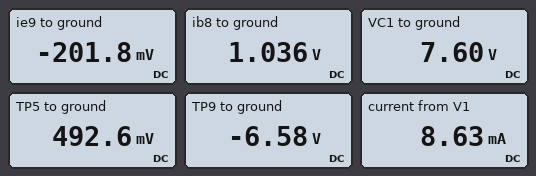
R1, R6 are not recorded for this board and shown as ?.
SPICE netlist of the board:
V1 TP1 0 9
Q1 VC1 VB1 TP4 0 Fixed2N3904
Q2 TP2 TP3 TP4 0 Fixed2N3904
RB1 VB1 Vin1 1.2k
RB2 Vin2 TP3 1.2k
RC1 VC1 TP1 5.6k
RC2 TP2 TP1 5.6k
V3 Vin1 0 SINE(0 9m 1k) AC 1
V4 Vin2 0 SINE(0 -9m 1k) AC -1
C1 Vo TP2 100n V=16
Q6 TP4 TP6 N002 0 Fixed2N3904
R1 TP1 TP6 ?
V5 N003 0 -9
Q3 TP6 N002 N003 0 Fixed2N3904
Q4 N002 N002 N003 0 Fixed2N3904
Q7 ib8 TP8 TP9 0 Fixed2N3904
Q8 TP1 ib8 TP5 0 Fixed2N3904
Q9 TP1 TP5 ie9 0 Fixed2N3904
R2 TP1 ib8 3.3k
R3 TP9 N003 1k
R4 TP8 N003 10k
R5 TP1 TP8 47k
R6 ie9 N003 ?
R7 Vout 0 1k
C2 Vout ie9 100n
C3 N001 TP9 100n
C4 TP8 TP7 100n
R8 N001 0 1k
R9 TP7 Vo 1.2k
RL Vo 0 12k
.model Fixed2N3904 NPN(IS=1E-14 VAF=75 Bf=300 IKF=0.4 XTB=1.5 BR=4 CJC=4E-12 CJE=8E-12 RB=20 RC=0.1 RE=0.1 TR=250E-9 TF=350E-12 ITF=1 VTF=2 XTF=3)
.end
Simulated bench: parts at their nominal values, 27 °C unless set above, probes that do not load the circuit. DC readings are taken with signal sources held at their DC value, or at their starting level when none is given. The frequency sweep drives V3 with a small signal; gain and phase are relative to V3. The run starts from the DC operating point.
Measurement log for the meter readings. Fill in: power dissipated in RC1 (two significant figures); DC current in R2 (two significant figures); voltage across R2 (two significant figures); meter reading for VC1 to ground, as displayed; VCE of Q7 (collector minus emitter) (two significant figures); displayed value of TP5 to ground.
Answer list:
350 µW
2.4 mA
8.0 V
7.60 V
7.6 V
492.6 mV
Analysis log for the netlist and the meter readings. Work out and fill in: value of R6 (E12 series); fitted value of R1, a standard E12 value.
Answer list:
1.8 kΩ
33 kΩ
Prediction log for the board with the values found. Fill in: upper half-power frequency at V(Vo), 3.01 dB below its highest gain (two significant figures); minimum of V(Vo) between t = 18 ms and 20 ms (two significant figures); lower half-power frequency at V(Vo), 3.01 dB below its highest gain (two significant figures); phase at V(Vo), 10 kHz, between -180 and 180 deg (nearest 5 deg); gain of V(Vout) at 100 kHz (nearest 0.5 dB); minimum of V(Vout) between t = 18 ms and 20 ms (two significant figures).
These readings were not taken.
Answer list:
1.2 MHz
-210 mV
85 Hz
0 deg
42.5 dB
-430 mV
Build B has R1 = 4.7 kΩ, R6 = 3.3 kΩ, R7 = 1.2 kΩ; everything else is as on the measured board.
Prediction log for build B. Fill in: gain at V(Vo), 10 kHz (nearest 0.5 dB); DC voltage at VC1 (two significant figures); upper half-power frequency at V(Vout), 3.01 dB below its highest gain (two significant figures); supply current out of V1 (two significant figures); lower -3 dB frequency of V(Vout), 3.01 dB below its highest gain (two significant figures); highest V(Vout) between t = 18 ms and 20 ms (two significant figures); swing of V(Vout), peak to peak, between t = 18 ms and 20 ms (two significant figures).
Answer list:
-4.5 dB
-640 mV
180 kHz
12 mA
2.0 kHz
12 mV
23 mV
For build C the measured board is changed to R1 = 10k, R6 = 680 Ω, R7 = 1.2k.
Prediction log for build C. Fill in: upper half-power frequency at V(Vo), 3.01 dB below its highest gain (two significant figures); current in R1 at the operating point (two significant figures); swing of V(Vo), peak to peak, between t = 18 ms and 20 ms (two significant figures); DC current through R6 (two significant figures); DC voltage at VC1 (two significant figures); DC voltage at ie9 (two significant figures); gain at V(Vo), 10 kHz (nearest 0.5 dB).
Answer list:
470 kHz
1.7 mA
1.3 V
13 mA
4.4 V
-250 mV
37.0 dB
